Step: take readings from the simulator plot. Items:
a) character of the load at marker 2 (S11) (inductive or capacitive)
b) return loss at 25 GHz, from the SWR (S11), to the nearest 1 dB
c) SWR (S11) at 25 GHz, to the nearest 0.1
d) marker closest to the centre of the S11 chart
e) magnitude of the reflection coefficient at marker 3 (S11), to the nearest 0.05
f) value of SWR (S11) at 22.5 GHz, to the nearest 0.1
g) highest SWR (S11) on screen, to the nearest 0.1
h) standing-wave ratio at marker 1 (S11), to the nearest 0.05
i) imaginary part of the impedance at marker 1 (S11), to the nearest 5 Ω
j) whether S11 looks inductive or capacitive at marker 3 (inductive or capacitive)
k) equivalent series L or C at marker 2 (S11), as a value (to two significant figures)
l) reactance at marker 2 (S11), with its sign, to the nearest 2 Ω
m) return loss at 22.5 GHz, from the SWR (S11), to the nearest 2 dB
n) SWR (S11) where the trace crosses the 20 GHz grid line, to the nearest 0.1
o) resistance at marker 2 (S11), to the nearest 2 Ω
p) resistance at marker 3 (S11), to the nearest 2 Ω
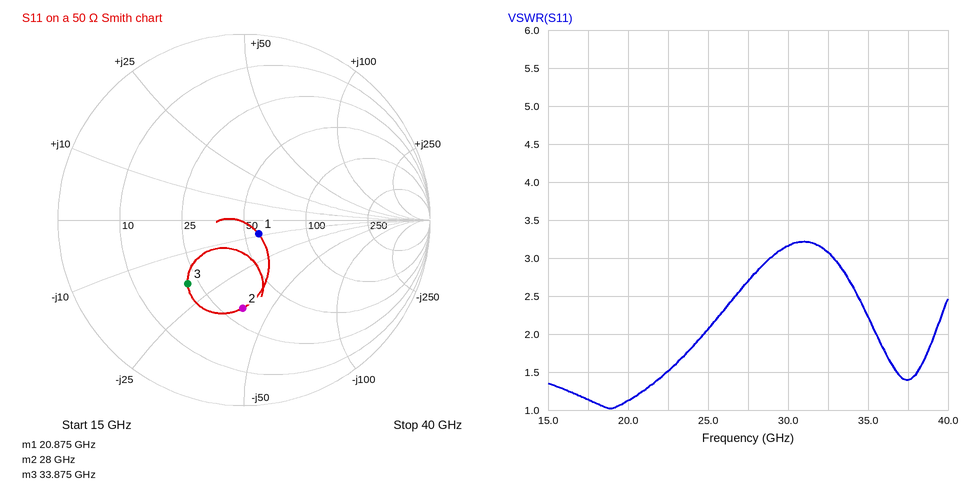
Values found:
capacitive
9 dB
2.1
marker 1
0.45
1.5
3.2
1.25
-10 Ω
capacitive
150 fF
-38 Ω
14 dB
1.1
32 Ω
22 Ω
